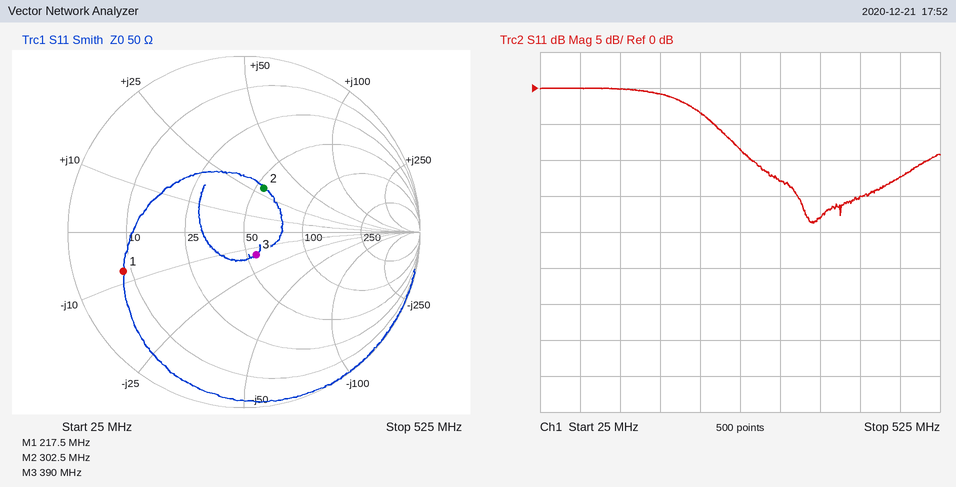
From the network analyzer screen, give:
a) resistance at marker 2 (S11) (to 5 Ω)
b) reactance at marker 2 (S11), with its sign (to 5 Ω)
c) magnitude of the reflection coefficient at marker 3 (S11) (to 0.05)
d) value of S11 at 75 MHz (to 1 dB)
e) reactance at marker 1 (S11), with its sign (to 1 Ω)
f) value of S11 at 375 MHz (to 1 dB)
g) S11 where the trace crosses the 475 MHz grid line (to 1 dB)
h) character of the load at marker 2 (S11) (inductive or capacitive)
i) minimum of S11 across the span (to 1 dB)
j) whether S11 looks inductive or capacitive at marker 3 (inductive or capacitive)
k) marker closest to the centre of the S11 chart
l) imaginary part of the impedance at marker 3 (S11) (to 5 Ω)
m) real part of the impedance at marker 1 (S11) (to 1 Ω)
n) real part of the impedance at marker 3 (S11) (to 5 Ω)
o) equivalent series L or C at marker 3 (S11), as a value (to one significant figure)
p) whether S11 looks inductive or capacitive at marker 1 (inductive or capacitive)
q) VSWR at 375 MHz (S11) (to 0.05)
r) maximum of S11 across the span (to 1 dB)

55 Ω
+30 Ω
0.15
0 dB
-8 Ω
-18 dB
-12 dB
inductive
-19 dB
capacitive
marker 3
-15 Ω
8 Ω
55 Ω
30 pF
capacitive
1.30
0 dB
